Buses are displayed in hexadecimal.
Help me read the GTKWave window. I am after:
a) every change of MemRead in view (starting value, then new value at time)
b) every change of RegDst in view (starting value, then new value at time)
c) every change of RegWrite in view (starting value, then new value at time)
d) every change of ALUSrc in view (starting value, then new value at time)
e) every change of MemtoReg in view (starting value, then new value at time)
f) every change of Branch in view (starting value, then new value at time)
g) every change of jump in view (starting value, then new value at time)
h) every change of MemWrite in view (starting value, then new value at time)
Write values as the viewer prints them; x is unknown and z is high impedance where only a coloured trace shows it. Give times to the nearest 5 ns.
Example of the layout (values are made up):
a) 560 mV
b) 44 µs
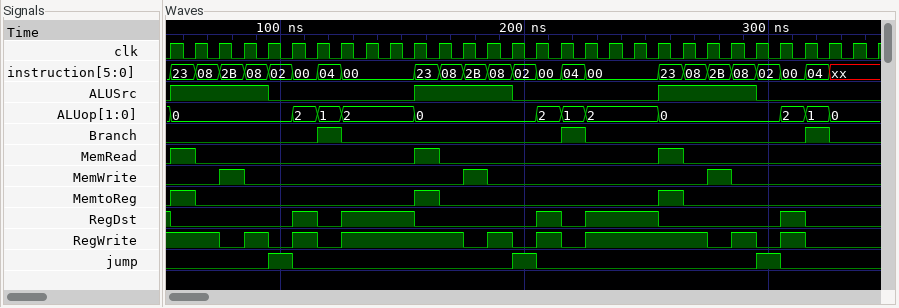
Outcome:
a) 0, 1 at 55 ns, 0 at 65 ns, 1 at 155 ns, 0 at 165 ns, 1 at 255 ns, 0 at 265 ns
b) 1, 0 at 55 ns, 1 at 105 ns, 0 at 115 ns, 1 at 125 ns, 0 at 155 ns, 1 at 205 ns, 0 at 215 ns, 1 at 225 ns, 0 at 255 ns, 1 at 305 ns, 0 at 315 ns
c) 1, 0 at 75 ns, 1 at 85 ns, 0 at 95 ns, 1 at 105 ns, 0 at 115 ns, 1 at 125 ns, 0 at 175 ns, 1 at 185 ns, 0 at 195 ns, 1 at 205 ns, 0 at 215 ns, 1 at 225 ns, 0 at 275 ns, 1 at 285 ns, 0 at 295 ns, 1 at 305 ns, 0 at 315 ns
d) 0, 1 at 55 ns, 0 at 95 ns, 1 at 155 ns, 0 at 195 ns, 1 at 255 ns, 0 at 295 ns
e) 0, 1 at 55 ns, 0 at 65 ns, 1 at 155 ns, 0 at 165 ns, 1 at 255 ns, 0 at 265 ns
f) 0, 1 at 115 ns, 0 at 125 ns, 1 at 215 ns, 0 at 225 ns, 1 at 315 ns, 0 at 325 ns
g) 0, 1 at 95 ns, 0 at 105 ns, 1 at 195 ns, 0 at 205 ns, 1 at 295 ns, 0 at 305 ns
h) 0, 1 at 75 ns, 0 at 85 ns, 1 at 175 ns, 0 at 185 ns, 1 at 275 ns, 0 at 285 ns
